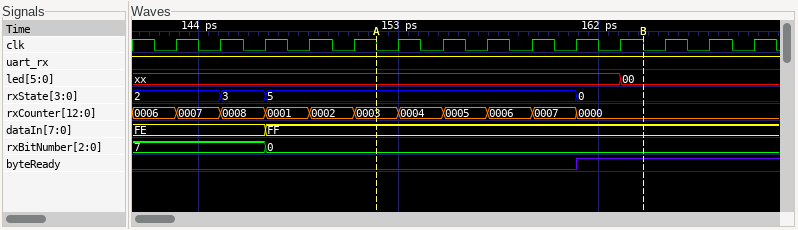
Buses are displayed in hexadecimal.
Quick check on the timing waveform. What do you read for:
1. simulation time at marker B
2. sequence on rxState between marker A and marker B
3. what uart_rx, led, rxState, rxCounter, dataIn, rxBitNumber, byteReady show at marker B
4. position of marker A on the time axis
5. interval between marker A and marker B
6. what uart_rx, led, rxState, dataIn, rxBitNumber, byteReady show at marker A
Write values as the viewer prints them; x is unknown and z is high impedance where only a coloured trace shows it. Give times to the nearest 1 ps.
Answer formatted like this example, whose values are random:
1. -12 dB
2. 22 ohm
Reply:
1. 164 ps
2. 5, 0
3. uart_rx=1, led=00, rxState=0, rxCounter=0000, dataIn=FF, rxBitNumber=0, byteReady=1
4. 152 ps
5. 12 ps
6. uart_rx=1, led=xx, rxState=5, dataIn=FF, rxBitNumber=0, byteReady=0
